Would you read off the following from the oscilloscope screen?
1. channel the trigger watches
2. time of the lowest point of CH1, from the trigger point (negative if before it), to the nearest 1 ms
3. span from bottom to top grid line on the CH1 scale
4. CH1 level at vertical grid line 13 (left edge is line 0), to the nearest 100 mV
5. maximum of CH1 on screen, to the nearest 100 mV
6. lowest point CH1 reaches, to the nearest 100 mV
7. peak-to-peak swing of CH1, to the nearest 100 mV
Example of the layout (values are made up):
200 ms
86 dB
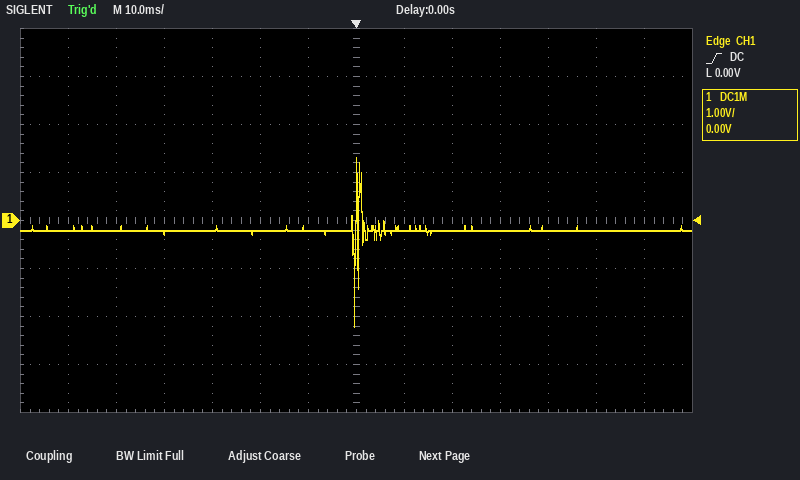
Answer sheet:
CH1
0 ms
8 V
-200 mV
1.3 V
-2.2 V
3.5 V
